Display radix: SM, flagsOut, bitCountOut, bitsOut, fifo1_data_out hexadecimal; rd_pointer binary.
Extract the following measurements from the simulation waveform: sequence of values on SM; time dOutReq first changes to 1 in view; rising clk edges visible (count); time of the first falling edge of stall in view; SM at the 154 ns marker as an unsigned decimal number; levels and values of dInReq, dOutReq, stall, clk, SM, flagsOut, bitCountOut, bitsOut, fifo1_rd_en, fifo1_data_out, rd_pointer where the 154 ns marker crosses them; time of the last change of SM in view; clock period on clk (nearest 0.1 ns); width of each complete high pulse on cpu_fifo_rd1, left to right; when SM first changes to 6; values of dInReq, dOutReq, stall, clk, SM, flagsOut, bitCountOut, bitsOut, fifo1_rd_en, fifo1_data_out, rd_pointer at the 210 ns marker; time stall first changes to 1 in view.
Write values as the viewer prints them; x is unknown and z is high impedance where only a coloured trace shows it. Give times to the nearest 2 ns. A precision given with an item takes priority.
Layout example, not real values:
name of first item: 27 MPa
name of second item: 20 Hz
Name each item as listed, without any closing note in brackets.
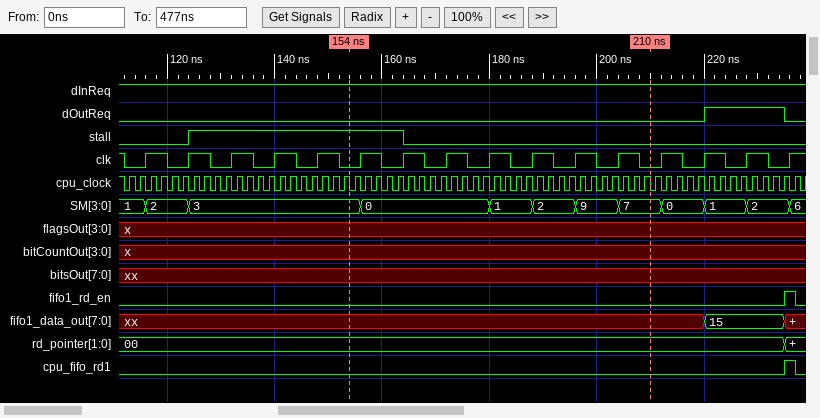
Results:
sequence of values on SM: 1, 2, 3, 0, 1, 2, 9, 7, 0, 1, 2, 6
time dOutReq first changes to 1 in view: 220 ns
rising clk edges visible: 16
time of the first falling edge of stall in view: 164 ns
SM at the 154 ns marker as an unsigned decimal number: 3
levels and values of dInReq, dOutReq, stall, clk, SM, flagsOut, bitCountOut, bitsOut, fifo1_rd_en, fifo1_data_out, rd_pointer where the 154 ns marker crosses them: dInReq=1, dOutReq=0, stall=1, clk=0, SM=3, flagsOut=x, bitCountOut=x, bitsOut=xx, fifo1_rd_en=0, fifo1_data_out=xx, rd_pointer=00
time of the last change of SM in view: 236 ns
clock period on clk: 8 ns
width of each complete high pulse on cpu_fifo_rd1, left to right: 2 ns
when SM first changes to 6: 236 ns
values of dInReq, dOutReq, stall, clk, SM, flagsOut, bitCountOut, bitsOut, fifo1_rd_en, fifo1_data_out, rd_pointer at the 210 ns marker: dInReq=1, dOutReq=0, stall=0, clk=0, SM=7, flagsOut=x, bitCountOut=x, bitsOut=xx, fifo1_rd_en=0, fifo1_data_out=xx, rd_pointer=00
time stall first changes to 1 in view: 124 ns
